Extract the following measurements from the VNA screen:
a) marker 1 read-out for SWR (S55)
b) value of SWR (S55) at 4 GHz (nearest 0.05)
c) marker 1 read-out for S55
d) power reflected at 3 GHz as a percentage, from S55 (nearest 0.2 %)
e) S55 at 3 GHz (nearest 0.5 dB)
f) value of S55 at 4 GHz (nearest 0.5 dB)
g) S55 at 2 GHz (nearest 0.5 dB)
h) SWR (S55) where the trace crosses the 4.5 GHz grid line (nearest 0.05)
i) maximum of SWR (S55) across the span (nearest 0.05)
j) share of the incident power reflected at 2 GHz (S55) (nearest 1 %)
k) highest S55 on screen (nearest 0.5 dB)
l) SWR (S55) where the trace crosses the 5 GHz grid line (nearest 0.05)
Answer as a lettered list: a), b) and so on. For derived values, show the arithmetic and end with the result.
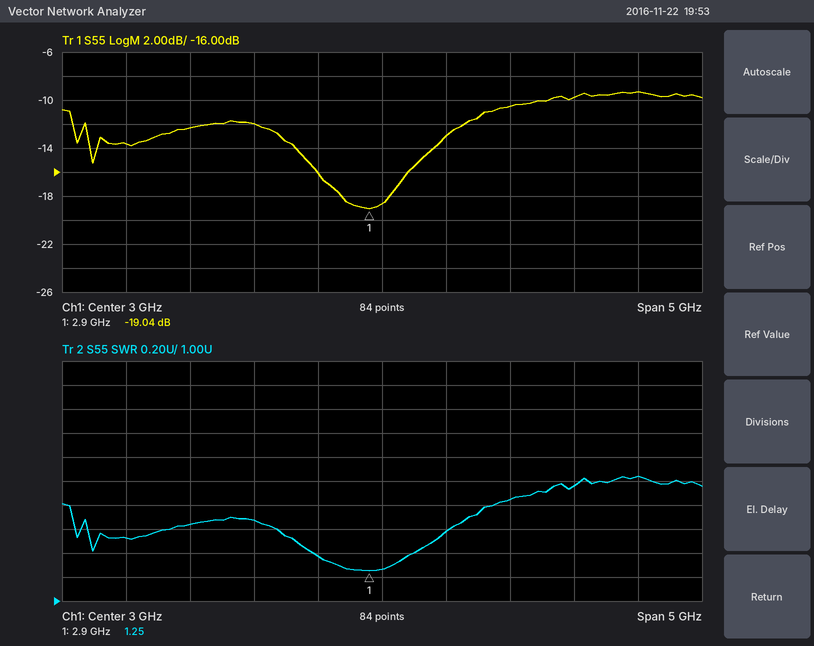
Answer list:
a) 1.25
b) 1.85
c) -19.04 dB
d) 10^(-18.5/10) ≈ 1.4 %
e) -18.5 dB
f) -10.5 dB
g) -12.0 dB
h) 1.95
i) 2.05
j) 10^(-12/10) ≈ 6 %
k) -9.5 dB
l) 2.05
